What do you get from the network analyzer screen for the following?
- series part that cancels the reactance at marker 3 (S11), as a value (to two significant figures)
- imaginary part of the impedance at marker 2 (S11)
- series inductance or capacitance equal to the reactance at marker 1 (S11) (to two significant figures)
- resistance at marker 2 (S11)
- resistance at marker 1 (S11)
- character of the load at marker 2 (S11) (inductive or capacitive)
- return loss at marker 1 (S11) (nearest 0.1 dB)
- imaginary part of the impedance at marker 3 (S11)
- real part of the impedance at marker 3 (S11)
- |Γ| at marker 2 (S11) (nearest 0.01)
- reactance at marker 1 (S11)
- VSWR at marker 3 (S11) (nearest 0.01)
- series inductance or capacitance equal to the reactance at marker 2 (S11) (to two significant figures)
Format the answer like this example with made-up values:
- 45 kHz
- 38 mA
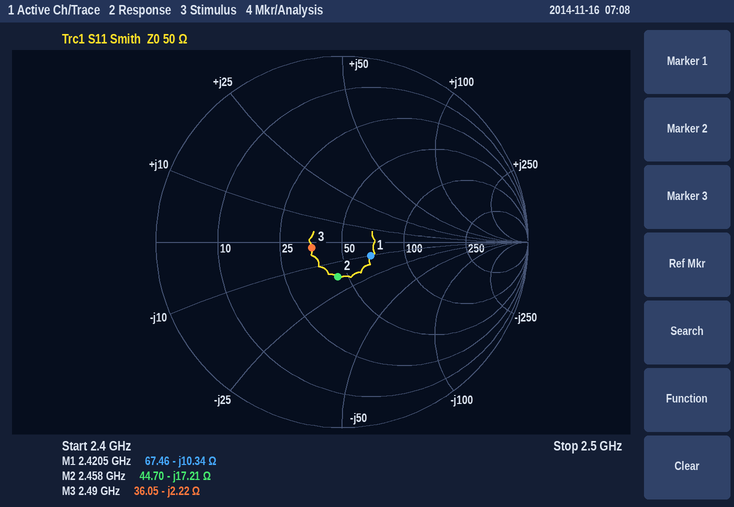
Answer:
- 140 pH
- -17.21 Ω
- 6.4 pF
- 44.70 Ω
- 67.46 Ω
- capacitive
- 15.3 dB
- -2.22 Ω
- 36.05 Ω
- 0.19
- -10.34 Ω
- 1.39
- 3.8 pF
